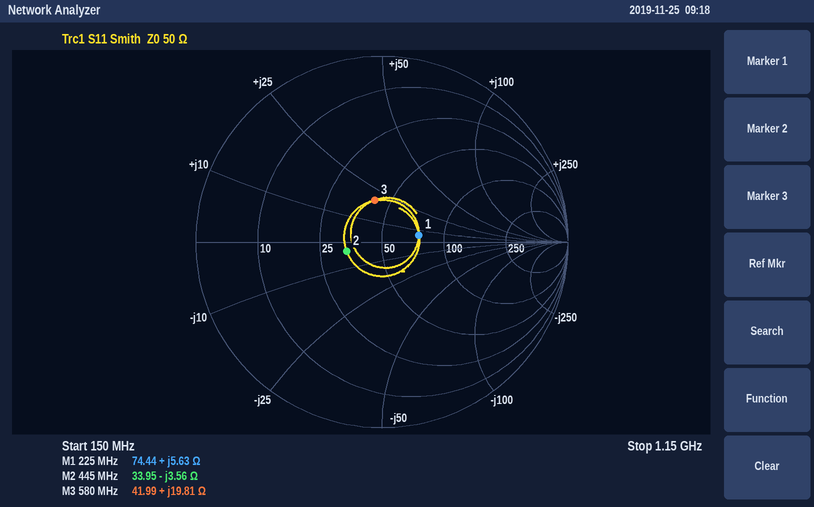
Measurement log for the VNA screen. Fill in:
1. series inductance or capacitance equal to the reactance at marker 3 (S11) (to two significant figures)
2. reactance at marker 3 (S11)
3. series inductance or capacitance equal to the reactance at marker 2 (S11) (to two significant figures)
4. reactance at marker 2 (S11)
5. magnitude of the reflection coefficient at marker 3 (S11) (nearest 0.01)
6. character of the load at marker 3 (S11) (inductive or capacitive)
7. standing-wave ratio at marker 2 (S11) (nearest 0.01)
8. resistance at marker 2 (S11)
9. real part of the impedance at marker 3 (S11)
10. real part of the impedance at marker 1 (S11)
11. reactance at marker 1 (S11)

5.4 nH
+19.81 Ω
100 pF
-3.56 Ω
0.23
inductive
1.49
33.95 Ω
41.99 Ω
74.44 Ω
+5.63 Ω
